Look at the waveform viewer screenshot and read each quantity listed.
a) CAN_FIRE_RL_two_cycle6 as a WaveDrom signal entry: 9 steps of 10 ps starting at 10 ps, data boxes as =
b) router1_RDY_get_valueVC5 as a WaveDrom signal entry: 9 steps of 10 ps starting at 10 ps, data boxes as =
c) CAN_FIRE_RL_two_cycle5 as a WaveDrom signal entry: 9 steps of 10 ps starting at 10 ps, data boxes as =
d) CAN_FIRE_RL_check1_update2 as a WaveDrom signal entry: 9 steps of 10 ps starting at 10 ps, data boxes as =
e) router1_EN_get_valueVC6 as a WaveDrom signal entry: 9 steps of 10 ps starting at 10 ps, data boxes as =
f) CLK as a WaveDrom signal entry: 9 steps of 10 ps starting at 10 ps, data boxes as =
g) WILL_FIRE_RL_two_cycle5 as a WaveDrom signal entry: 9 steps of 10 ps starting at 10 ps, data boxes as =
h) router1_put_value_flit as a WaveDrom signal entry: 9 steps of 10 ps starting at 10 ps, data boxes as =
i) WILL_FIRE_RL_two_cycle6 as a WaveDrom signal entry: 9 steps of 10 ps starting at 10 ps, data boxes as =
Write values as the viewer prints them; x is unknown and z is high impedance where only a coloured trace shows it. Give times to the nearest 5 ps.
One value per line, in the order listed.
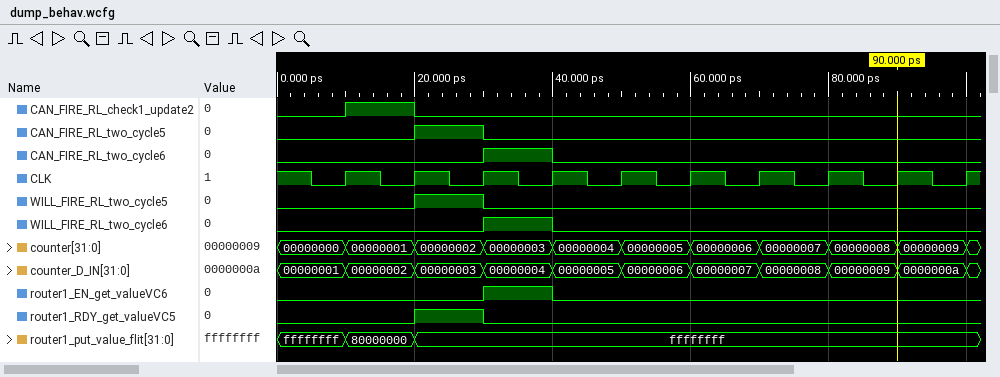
{name: 'CAN_FIRE_RL_two_cycle6', wave: '0.10.....'}
{name: 'router1_RDY_get_valueVC5', wave: '010......'}
{name: 'CAN_FIRE_RL_two_cycle5', wave: '010......'}
{name: 'CAN_FIRE_RL_check1_update2', wave: '10.......'}
{name: 'router1_EN_get_valueVC6', wave: '0.10.....'}
{name: 'CLK', wave: 'p........'}
{name: 'WILL_FIRE_RL_two_cycle5', wave: '010......'}
{name: 'router1_put_value_flit', wave: '==.......', data: '80000000 ffffffff'}
{name: 'WILL_FIRE_RL_two_cycle6', wave: '0.10.....'}
